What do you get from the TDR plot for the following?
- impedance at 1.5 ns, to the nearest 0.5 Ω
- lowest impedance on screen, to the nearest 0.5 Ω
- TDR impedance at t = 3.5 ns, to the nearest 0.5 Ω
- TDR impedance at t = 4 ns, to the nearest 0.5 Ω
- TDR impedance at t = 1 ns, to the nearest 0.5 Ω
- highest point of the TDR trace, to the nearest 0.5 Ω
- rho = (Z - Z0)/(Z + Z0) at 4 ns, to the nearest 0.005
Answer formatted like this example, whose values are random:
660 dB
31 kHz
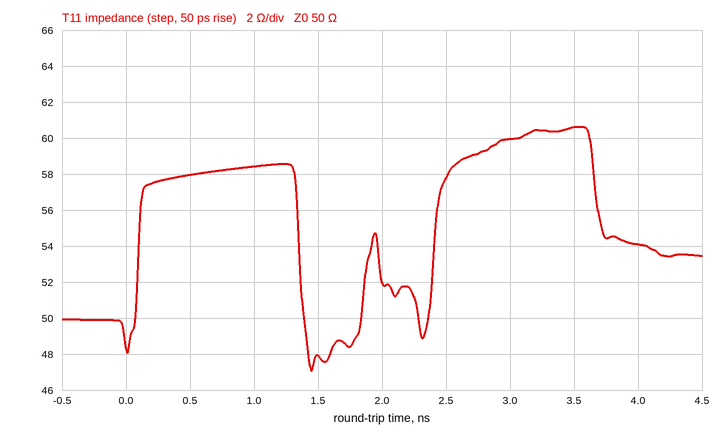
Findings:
48.0 Ω
47.0 Ω
60.5 Ω
54.0 Ω
58.5 Ω
60.5 Ω
+0.040
